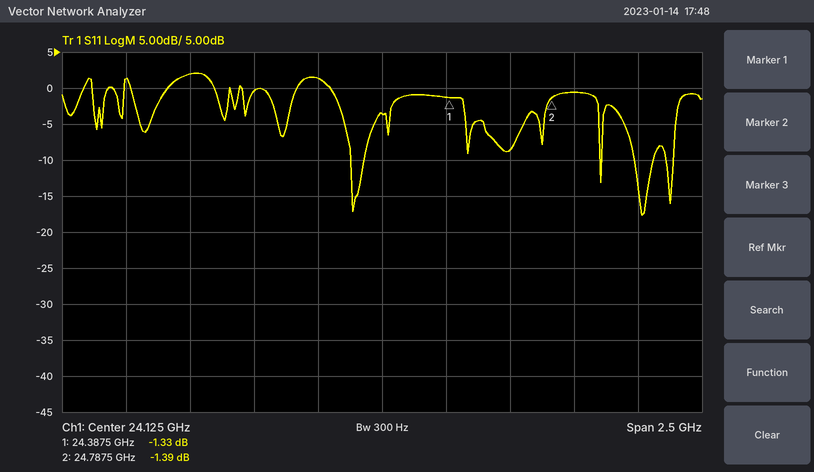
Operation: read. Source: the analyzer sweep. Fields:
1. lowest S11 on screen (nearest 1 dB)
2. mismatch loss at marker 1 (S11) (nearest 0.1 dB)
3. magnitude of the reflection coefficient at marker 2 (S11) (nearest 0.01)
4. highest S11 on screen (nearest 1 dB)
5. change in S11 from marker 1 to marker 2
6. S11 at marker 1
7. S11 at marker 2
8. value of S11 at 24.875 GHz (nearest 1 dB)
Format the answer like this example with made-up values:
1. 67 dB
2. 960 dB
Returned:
1. -18 dB
2. 5.8 dB
3. 0.85
4. 2 dB
5. -0.06 dB
6. -1.33 dB
7. -1.39 dB
8. -1 dB
